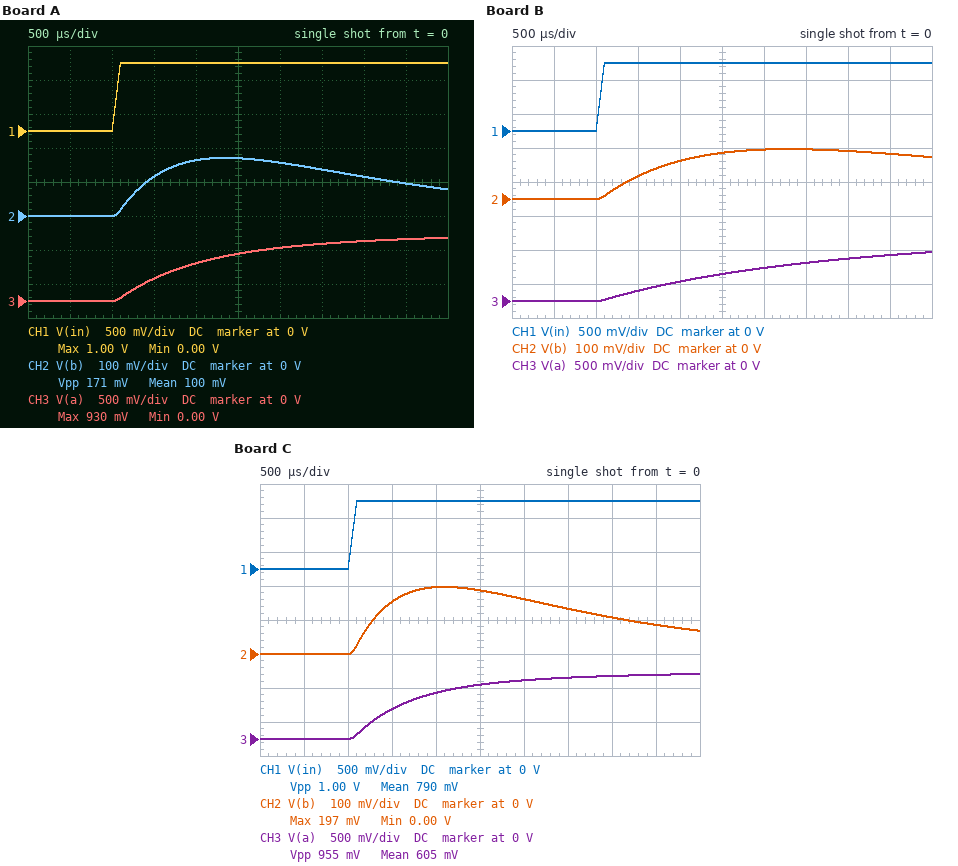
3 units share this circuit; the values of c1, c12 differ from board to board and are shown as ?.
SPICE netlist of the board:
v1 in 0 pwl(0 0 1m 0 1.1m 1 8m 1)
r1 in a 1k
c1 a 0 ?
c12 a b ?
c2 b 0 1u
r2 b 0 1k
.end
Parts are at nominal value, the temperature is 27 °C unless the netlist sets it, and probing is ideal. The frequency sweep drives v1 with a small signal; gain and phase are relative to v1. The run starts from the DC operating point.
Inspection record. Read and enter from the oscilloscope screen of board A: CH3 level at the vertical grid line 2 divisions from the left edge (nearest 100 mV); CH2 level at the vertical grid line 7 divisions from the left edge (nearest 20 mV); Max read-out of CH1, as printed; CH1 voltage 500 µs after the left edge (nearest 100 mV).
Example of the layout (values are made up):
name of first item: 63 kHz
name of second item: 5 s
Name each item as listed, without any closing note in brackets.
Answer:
CH3 level at the vertical grid line 2 divisions from the left edge: 0 V
CH2 level at the vertical grid line 7 divisions from the left edge: 140 mV
Max read-out of CH1, as printed: 1.00 V
CH1 voltage 500 µs after the left edge: 0 V
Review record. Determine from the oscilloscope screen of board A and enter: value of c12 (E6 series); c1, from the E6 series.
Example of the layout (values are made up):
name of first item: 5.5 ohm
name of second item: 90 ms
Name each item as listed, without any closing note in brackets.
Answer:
value of c12: 680 nF
c1, from the E6 series: 680 nF
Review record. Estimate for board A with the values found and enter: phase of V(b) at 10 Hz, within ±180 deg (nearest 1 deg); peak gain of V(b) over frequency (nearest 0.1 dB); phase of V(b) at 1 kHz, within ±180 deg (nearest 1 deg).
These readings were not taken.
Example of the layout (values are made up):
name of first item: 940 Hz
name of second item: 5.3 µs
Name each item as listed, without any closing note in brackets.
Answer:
phase of V(b) at 10 Hz, within ±180 deg: 79 deg
peak gain of V(b) over frequency: -13.0 dB
phase of V(b) at 1 kHz, within ±180 deg: -75 deg
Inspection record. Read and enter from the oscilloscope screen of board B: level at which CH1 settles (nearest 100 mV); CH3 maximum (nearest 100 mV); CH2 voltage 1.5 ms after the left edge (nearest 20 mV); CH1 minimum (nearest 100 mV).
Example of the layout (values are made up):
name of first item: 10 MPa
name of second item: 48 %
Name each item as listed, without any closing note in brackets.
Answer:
level at which CH1 settles: 1.0 V
CH3 maximum: 700 mV
CH2 voltage 1.5 ms after the left edge: 60 mV
CH1 minimum: 0 V
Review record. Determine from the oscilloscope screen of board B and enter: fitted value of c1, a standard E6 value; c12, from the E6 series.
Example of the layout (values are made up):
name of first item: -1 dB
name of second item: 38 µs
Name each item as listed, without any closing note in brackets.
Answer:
fitted value of c1, a standard E6 value: 2.2 µF
c12, from the E6 series: 1 µF
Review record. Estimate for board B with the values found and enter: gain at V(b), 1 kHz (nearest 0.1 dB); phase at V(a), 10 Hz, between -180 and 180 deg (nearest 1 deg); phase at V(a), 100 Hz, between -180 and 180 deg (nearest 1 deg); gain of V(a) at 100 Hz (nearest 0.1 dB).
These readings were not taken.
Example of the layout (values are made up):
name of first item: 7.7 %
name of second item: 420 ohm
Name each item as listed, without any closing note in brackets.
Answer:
gain at V(b), 1 kHz: -30.7 dB
phase at V(a), 10 Hz, between -180 and 180 deg: -11 deg
phase at V(a), 100 Hz, between -180 and 180 deg: -58 deg
gain of V(a) at 100 Hz: -6.7 dB
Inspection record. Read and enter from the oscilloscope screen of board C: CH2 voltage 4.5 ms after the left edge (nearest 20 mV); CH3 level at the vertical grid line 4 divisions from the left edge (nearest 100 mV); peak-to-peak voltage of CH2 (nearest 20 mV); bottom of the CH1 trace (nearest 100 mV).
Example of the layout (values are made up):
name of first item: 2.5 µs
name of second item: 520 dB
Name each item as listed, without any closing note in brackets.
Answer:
CH2 voltage 4.5 ms after the left edge: 80 mV
CH3 level at the vertical grid line 4 divisions from the left edge: 700 mV
peak-to-peak voltage of CH2: 200 mV
bottom of the CH1 trace: 0 V
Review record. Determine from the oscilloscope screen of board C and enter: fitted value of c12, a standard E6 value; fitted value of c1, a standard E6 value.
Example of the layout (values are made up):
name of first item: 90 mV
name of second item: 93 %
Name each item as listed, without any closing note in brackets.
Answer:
fitted value of c12, a standard E6 value: 680 nF
fitted value of c1, a standard E6 value: 330 nF
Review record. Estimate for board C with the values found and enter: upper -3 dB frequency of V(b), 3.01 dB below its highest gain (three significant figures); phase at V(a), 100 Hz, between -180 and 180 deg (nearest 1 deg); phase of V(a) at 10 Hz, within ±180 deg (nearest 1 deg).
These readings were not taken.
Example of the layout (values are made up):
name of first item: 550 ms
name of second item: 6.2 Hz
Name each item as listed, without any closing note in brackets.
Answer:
upper -3 dB frequency of V(b), 3.01 dB below its highest gain: 398 Hz
phase at V(a), 100 Hz, between -180 and 180 deg: -27 deg
phase of V(a) at 10 Hz, within ±180 deg: -4 deg
